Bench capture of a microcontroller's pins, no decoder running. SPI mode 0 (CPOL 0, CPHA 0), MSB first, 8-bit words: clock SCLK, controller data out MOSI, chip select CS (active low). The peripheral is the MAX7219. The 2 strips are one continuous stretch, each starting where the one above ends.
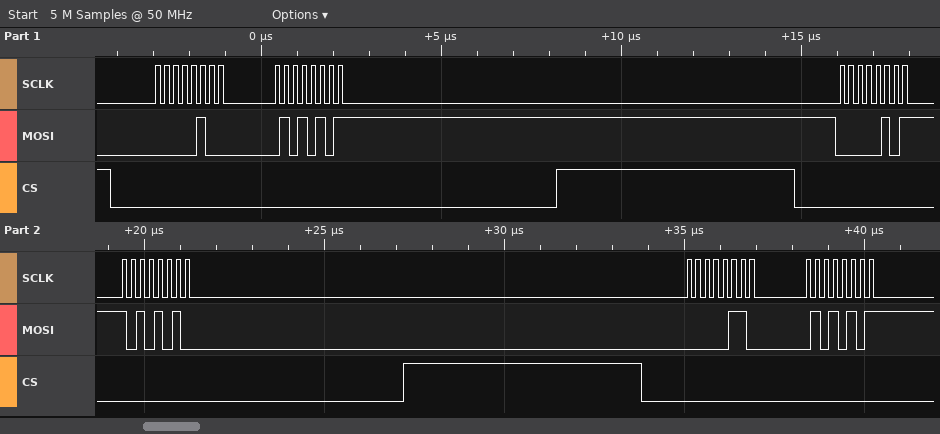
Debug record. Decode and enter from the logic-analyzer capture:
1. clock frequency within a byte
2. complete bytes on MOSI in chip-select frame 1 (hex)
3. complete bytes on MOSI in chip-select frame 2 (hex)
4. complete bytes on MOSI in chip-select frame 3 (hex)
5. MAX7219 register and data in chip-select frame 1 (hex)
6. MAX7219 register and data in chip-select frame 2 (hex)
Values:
4 MHz
04 55
05 AA
06 55
register 0x4, data 0x55
register 0x5, data 0xAA
